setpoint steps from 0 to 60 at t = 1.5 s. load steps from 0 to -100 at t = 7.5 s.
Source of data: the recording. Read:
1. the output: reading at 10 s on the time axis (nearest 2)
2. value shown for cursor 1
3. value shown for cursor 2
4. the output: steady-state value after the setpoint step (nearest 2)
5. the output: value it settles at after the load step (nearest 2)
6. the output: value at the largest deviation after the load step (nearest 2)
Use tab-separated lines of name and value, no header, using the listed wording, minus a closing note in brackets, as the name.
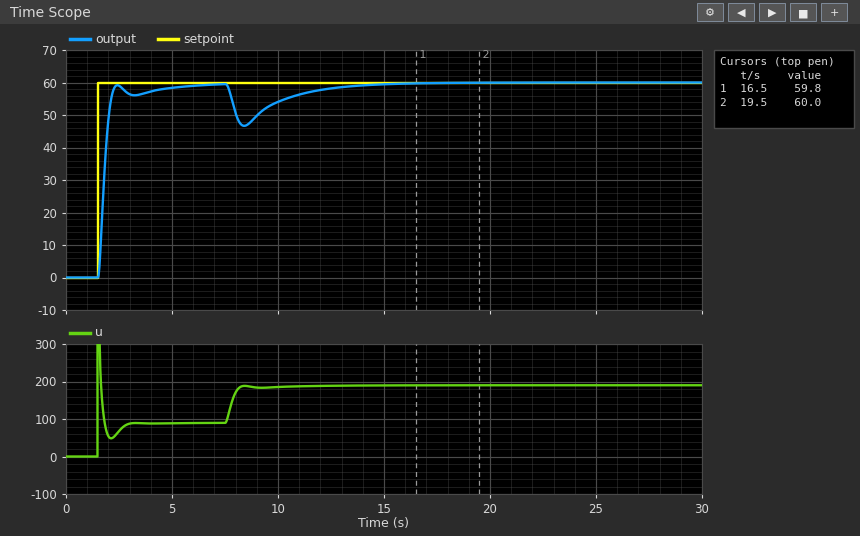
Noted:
the output: reading at 10 s on the time axis	54
value shown for cursor 1	59.8
value shown for cursor 2	60.0
the output: steady-state value after the setpoint step	60
the output: value it settles at after the load step	60
the output: value at the largest deviation after the load step	46
